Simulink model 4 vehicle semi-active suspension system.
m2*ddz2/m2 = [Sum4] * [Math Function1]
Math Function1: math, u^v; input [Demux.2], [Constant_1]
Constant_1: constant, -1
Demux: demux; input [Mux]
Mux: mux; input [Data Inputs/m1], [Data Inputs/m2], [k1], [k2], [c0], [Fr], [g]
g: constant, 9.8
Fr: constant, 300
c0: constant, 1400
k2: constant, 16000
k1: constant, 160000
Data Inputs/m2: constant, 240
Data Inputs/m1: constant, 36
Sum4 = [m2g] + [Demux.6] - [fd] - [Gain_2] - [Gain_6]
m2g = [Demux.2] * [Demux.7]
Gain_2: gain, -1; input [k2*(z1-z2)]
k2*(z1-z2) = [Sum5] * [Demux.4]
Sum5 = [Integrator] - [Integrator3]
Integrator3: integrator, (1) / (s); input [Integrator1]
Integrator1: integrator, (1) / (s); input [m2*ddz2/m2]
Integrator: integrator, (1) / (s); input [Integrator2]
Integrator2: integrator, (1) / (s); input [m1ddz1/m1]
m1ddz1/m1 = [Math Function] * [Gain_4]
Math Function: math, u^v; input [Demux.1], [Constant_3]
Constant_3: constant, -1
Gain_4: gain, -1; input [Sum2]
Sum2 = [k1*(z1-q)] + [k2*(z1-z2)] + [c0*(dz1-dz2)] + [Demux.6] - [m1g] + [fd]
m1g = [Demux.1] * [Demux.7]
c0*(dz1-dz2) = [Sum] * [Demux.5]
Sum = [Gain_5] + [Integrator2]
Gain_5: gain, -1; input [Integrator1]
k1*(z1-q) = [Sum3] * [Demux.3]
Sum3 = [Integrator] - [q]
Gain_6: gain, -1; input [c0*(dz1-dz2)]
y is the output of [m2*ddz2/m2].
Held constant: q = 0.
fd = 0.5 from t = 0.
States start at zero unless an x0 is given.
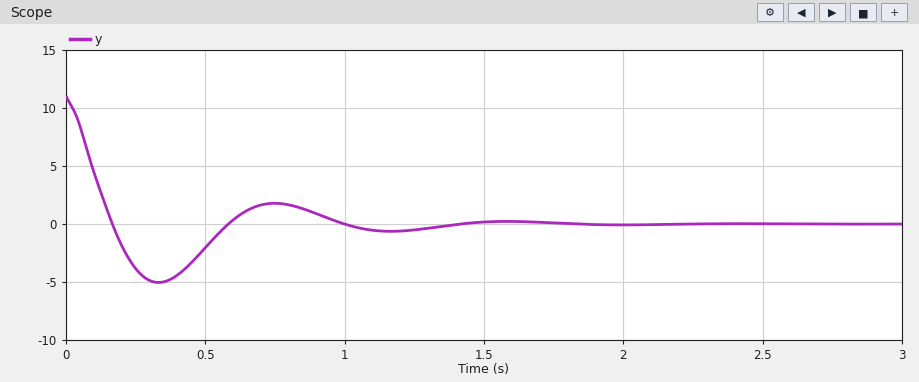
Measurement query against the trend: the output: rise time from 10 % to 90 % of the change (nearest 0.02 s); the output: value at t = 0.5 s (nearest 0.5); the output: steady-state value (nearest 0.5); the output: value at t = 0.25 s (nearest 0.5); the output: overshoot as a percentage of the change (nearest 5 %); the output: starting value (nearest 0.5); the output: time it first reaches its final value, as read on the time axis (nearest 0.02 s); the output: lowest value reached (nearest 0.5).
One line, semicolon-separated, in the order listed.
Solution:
0.12 s; -2.0; 0.0; -4.0; 45 %; 11.0; 0.16 s; -5.0
